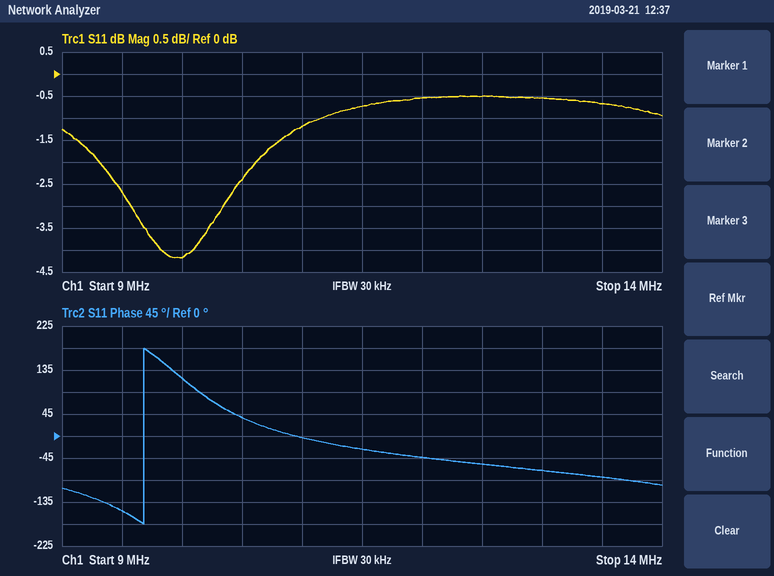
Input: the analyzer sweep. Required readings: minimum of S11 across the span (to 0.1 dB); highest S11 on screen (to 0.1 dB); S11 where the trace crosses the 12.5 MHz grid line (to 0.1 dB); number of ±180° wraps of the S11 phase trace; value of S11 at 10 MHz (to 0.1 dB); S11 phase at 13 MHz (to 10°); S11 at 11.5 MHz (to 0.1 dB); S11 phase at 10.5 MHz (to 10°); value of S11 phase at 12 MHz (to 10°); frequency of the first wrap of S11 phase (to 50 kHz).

-4.2 dB
-0.5 dB
-0.5 dB
1
-4.2 dB
-70°
-0.7 dB
40°
-40°
9.70 MHz
